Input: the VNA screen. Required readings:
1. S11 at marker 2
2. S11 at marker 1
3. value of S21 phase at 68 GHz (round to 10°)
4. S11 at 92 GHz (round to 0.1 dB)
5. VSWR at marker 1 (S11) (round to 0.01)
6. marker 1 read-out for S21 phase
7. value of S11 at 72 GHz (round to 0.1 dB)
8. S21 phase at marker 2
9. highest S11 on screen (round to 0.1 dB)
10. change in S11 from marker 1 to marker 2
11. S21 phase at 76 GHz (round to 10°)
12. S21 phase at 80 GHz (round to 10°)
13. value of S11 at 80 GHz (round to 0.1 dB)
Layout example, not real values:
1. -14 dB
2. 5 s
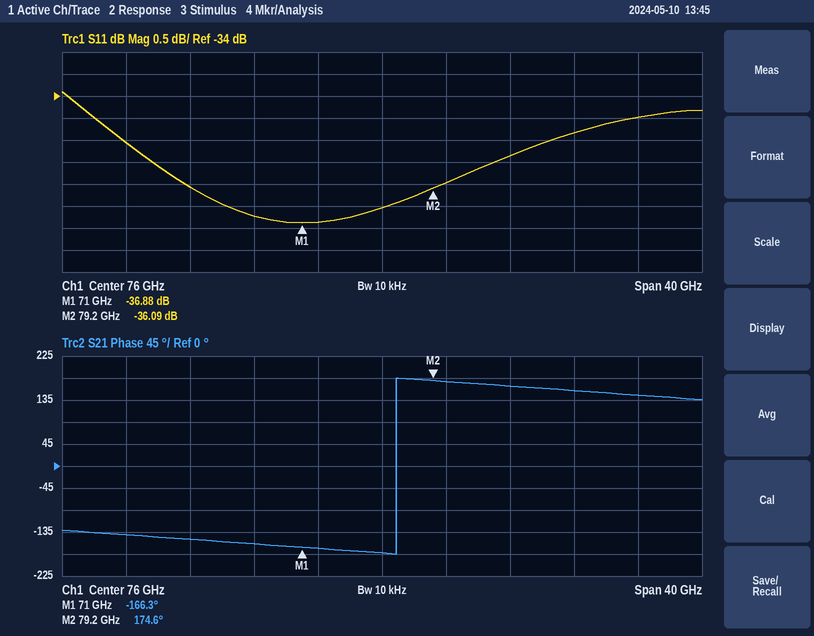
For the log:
1. -36.09 dB
2. -36.88 dB
3. -160°
4. -34.5 dB
5. 1.03
6. -166.3°
7. -36.9 dB
8. 174.6°
9. -33.9 dB
10. 0.79 dB
11. -180°
12. 170°
13. -36.0 dB
